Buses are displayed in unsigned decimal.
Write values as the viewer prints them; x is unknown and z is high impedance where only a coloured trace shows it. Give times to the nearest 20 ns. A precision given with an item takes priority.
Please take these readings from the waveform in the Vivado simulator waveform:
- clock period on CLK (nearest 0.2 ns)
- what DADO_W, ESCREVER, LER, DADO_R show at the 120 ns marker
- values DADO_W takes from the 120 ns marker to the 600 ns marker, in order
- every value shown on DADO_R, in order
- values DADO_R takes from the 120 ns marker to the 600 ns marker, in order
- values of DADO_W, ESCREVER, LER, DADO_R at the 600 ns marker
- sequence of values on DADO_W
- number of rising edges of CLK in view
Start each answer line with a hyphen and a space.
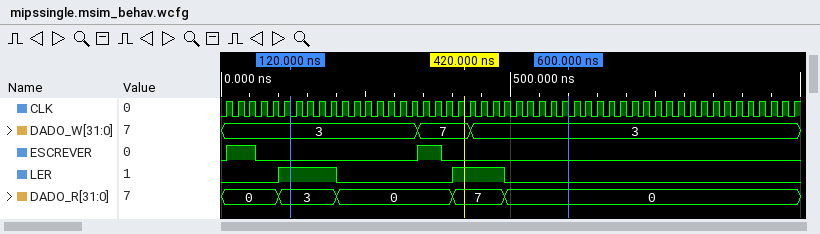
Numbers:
- 20 ns
- DADO_W=3, ESCREVER=0, LER=1, DADO_R=3
- 3, 7, 3
- 0, 3, 0, 7, 0
- 3, 0, 7, 0
- DADO_W=3, ESCREVER=0, LER=0, DADO_R=0
- 3, 7, 3
- 50
